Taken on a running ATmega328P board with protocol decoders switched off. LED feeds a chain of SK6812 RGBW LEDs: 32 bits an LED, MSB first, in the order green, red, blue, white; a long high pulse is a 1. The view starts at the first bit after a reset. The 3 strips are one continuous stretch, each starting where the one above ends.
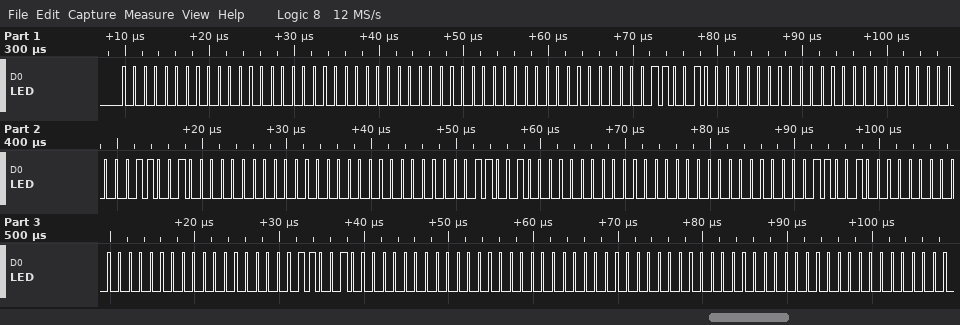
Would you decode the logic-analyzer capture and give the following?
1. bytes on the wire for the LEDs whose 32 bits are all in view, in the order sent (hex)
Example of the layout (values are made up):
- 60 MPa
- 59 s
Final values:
- 00 00 00 00 00 00 32 00 00 00 32 00 00 00 32 00 00 00 32 00 00 00 32 00 00 00 00 00
